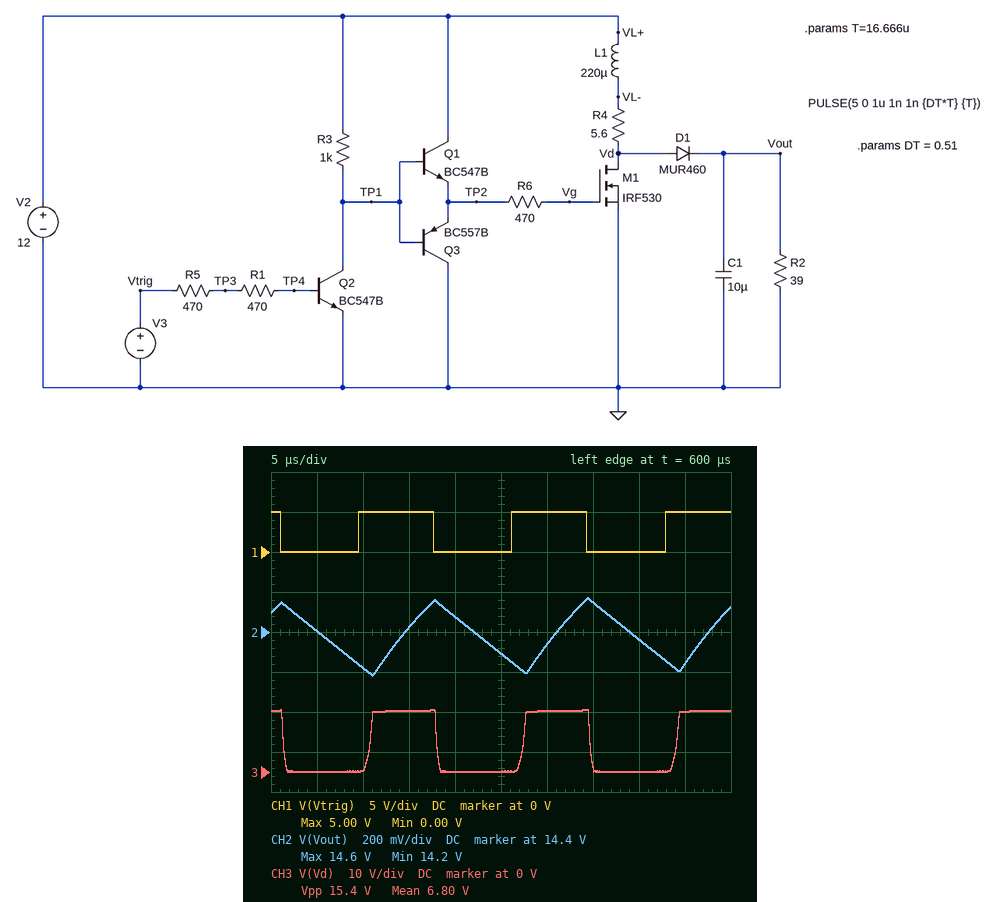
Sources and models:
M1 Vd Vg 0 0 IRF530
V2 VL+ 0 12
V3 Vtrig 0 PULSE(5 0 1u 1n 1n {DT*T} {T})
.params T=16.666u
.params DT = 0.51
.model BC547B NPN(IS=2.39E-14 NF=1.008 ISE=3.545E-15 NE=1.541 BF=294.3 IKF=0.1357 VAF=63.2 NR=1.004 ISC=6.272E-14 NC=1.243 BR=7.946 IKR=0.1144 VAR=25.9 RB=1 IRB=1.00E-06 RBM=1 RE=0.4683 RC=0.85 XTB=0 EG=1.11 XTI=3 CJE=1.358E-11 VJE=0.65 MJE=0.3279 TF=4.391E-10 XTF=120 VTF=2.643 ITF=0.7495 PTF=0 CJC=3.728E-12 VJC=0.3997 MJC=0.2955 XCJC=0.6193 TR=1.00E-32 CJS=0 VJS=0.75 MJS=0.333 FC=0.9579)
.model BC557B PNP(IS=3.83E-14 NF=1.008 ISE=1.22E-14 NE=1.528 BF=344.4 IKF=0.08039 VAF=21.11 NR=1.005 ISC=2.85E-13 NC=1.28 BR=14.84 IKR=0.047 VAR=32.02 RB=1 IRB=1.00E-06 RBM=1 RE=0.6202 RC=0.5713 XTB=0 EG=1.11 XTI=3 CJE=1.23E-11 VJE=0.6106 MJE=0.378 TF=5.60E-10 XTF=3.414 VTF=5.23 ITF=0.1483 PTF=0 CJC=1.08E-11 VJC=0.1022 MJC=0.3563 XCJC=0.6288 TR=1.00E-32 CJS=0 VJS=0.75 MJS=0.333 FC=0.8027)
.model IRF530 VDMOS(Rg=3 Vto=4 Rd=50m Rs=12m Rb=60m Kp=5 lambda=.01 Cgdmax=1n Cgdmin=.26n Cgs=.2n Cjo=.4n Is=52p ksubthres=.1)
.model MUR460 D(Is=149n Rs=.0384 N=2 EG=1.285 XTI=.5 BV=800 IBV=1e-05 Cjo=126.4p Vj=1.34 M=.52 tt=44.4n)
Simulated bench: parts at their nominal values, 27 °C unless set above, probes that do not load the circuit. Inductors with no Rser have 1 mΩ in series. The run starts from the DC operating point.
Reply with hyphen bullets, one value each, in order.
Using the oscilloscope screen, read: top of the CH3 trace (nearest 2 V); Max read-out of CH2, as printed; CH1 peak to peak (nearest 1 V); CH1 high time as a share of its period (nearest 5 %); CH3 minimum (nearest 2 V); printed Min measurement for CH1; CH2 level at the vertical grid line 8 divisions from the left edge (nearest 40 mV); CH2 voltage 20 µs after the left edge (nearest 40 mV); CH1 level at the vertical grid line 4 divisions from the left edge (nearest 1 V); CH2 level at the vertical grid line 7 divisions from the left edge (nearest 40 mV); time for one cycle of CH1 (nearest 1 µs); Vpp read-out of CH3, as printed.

- 16 V
- 14.6 V
- 5 V
- 50 %
- 0 V
- 0.00 V
- 14.36 V
- 14.48 V
- 0 V
- 14.56 V
- 17 µs
- 15.4 V
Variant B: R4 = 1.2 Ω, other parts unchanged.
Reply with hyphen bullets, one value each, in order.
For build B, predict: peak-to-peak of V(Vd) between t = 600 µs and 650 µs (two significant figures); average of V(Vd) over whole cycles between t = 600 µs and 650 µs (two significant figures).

- 23 V
- 10 V
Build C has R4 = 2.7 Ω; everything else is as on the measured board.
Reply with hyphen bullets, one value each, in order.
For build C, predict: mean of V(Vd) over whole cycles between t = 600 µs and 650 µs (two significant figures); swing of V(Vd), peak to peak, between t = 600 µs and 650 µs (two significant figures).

- 8.7 V
- 20 V
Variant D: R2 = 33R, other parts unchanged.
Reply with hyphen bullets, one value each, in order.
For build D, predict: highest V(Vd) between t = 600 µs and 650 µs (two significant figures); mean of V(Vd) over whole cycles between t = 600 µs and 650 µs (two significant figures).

- 14 V
- 6.3 V
